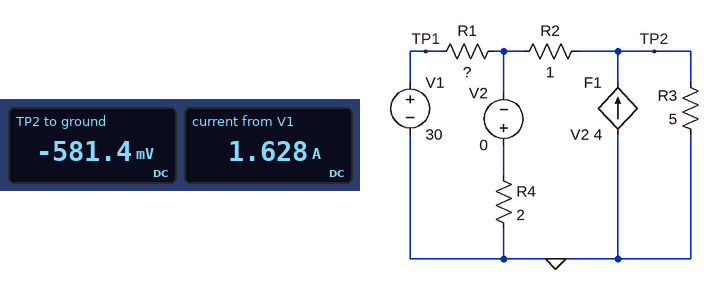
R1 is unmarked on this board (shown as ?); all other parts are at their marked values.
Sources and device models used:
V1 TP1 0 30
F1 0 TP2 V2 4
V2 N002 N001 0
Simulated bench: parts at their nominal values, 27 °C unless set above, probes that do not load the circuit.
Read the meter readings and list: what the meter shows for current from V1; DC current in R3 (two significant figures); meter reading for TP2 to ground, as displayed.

1.628 A
120 mA
-581.4 mV
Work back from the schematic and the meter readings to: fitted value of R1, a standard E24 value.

18 Ω
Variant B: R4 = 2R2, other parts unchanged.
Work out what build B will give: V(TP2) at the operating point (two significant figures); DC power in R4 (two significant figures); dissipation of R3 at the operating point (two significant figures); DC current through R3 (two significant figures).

-520 mV
260 mW
54 mW
100 mA
